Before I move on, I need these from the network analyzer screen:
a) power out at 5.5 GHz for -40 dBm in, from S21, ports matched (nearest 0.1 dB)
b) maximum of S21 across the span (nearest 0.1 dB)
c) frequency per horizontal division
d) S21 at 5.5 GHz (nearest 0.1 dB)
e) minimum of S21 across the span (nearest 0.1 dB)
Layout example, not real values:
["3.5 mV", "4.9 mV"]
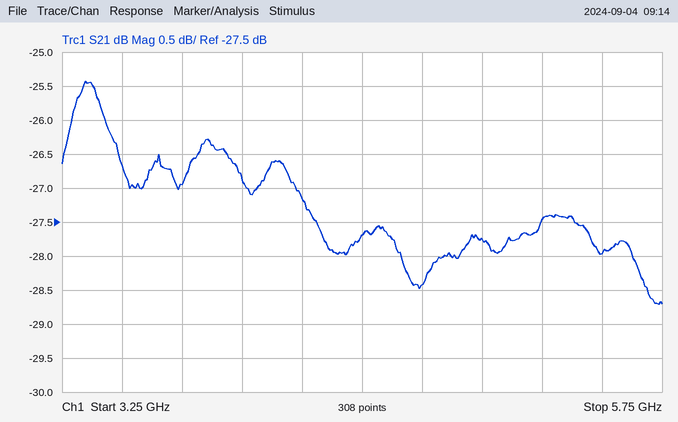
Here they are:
["-68.0 dBm", "-25.4 dB", "250 MHz", "-28.0 dB", "-28.7 dB"]
